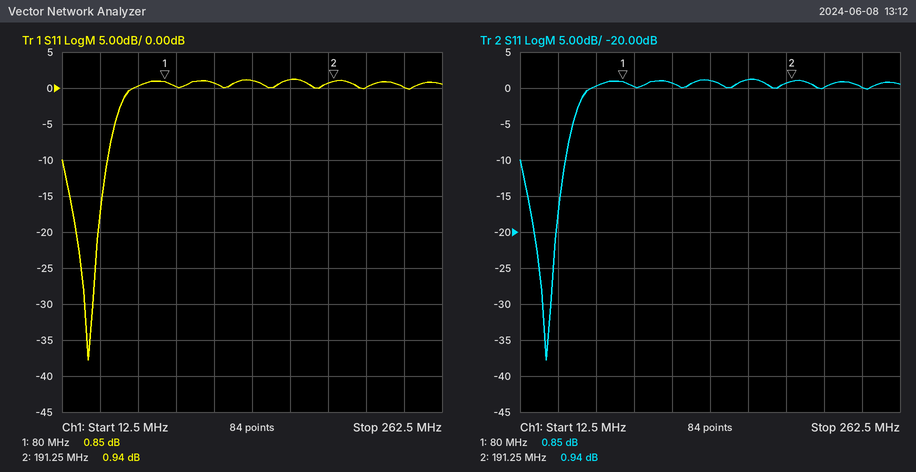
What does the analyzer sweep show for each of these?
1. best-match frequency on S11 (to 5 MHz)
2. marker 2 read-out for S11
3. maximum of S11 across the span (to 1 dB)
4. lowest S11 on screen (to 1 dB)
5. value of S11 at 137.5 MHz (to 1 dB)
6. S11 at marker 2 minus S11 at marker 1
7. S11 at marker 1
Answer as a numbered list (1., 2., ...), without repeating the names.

1. 30 MHz
2. 0.94 dB
3. 1 dB
4. -38 dB
5. 1 dB
6. 0.09 dB
7. 0.85 dB
